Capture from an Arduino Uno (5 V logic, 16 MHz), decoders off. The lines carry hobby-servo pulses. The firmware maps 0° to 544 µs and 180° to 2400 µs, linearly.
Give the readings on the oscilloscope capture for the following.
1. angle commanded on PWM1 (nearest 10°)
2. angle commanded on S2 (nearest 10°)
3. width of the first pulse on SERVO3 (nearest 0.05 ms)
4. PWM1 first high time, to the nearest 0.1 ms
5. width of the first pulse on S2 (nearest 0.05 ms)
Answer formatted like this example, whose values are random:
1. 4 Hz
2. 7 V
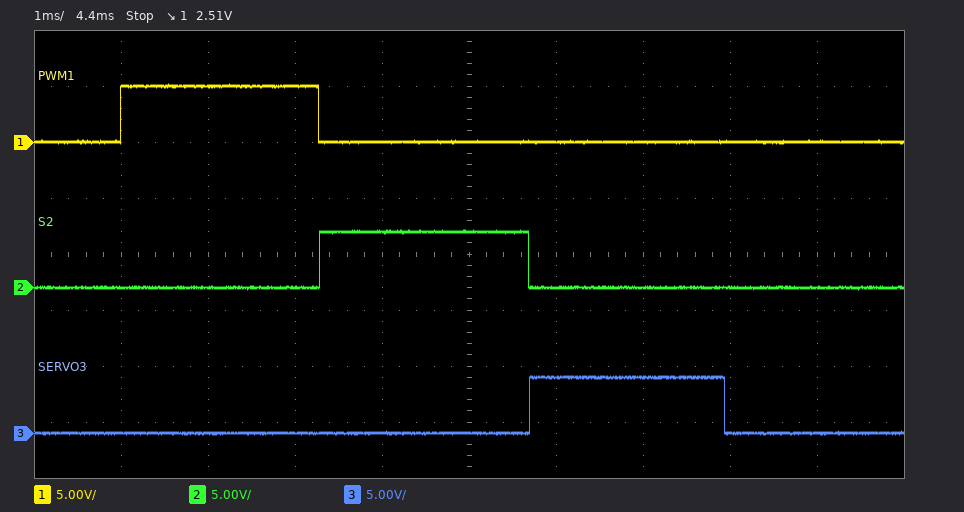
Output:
1. 170°
2. 180°
3. 2.25 ms
4. 2.3 ms
5. 2.40 ms
